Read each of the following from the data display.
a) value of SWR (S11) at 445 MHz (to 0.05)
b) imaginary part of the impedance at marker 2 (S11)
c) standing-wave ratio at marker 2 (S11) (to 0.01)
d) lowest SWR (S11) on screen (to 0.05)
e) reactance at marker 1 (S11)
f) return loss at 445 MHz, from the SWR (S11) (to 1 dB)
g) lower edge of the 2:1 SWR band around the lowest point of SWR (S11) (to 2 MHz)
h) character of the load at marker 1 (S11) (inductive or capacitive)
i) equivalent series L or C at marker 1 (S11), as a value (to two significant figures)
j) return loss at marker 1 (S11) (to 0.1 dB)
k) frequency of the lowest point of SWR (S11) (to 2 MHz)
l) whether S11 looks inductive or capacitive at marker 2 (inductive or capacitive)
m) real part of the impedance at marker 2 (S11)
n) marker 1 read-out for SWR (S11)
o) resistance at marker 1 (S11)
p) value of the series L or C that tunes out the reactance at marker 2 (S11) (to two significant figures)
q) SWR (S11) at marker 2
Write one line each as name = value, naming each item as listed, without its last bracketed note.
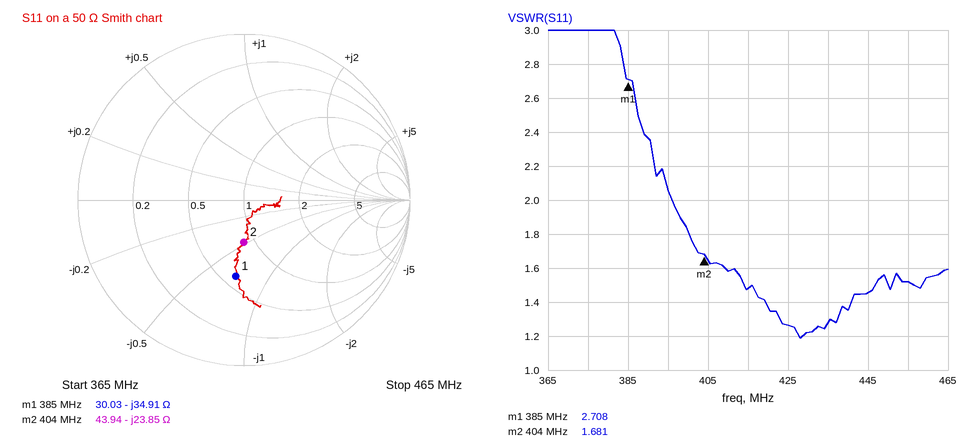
value of SWR (S11) at 445 MHz = 1.45
imaginary part of the impedance at marker 2 = -23.85 Ω
standing-wave ratio at marker 2 (S11) = 1.68
lowest SWR (S11) on screen = 1.20
reactance at marker 1 = -34.91 Ω
return loss at 445 MHz, from the SWR (S11) = 15 dB
lower edge of the 2:1 SWR band around the lowest point of SWR (S11) = 396 MHz
character of the load at marker 1 (S11) = capacitive
equivalent series L or C at marker 1 (S11), as a value = 12 pF
return loss at marker 1 (S11) = 6.7 dB
frequency of the lowest point of SWR (S11) = 428 MHz
whether S11 looks inductive or capacitive at marker 2 = capacitive
real part of the impedance at marker 2 = 43.94 Ω
marker 1 read-out for SWR = 2.708
resistance at marker 1 = 30.03 Ω
value of the series L or C that tunes out the reactance at marker 2 (S11) = 9.4 nH
SWR (S11) at marker 2 = 1.681
